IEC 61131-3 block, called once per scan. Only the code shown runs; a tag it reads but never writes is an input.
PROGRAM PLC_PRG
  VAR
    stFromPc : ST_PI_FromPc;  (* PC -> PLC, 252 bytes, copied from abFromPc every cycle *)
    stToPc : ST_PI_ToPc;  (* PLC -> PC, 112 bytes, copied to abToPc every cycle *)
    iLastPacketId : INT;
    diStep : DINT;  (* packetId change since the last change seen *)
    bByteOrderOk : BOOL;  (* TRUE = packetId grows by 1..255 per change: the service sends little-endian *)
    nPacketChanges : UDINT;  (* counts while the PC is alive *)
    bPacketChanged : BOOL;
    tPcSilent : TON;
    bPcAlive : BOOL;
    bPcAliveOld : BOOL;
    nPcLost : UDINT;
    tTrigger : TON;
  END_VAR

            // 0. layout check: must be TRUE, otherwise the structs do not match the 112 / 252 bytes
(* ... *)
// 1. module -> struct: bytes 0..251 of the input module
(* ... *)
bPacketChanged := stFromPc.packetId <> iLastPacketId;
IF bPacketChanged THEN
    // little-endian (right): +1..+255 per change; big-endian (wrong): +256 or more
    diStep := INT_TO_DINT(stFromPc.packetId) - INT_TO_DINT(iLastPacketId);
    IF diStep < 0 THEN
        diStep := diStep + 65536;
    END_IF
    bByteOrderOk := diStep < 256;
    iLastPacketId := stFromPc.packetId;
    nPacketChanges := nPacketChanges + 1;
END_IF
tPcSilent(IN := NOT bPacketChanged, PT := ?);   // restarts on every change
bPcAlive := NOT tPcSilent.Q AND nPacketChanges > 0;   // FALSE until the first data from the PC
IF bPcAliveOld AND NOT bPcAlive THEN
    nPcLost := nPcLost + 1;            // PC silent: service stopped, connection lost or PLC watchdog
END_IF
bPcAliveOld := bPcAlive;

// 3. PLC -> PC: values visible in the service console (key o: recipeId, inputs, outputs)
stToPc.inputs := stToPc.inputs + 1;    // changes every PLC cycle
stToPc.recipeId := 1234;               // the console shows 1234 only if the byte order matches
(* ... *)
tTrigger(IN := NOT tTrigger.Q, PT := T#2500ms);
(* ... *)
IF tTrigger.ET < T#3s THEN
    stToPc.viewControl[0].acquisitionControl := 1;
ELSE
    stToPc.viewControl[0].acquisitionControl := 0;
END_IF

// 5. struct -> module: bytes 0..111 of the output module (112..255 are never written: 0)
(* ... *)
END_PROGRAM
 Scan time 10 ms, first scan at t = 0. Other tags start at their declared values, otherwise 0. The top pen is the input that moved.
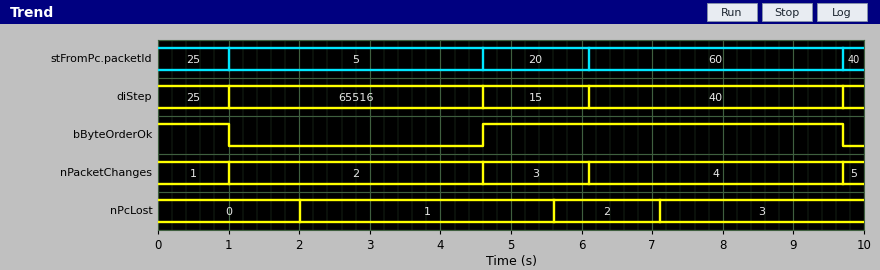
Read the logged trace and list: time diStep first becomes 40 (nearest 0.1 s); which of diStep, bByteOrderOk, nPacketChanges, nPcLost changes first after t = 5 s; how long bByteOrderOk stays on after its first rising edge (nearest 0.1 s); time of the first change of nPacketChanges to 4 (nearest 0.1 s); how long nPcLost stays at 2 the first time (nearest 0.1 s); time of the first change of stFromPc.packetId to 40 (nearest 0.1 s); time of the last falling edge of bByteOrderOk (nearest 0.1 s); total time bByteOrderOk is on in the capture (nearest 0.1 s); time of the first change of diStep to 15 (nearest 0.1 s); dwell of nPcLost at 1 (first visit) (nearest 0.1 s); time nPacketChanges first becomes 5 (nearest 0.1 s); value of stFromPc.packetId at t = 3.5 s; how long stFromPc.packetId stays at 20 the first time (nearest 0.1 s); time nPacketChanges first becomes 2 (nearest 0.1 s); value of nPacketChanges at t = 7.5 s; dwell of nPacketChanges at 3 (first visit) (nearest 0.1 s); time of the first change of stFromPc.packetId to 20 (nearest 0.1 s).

6.1 s
nPcLost
5.1 s
6.1 s
1.5 s
9.7 s
9.7 s
6.1 s
4.6 s
3.6 s
9.7 s
5
1.5 s
1.0 s
4
1.5 s
4.6 s
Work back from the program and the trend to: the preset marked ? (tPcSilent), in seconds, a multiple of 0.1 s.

1.0 s
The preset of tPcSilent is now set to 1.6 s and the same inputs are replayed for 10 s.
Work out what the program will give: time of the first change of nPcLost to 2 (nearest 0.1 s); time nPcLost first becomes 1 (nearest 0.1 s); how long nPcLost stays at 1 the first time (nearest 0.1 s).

7.7 s
2.6 s
5.1 s
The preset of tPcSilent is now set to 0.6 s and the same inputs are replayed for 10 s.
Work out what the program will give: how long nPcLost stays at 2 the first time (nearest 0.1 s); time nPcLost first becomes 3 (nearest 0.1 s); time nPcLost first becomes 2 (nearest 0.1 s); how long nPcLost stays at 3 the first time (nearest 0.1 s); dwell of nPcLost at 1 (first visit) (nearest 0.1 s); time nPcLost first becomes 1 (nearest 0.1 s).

3.6 s
5.2 s
1.6 s
1.5 s
1.0 s
0.6 s
